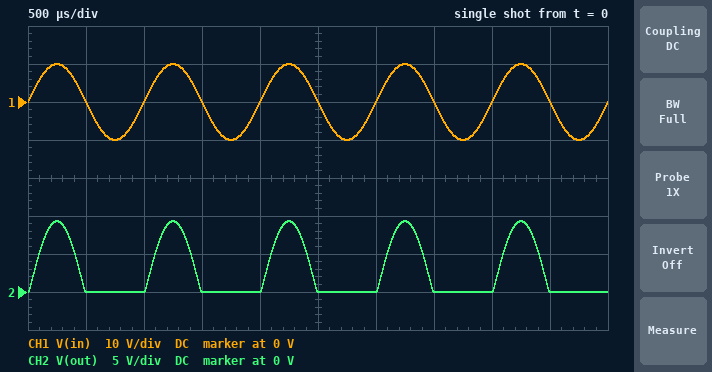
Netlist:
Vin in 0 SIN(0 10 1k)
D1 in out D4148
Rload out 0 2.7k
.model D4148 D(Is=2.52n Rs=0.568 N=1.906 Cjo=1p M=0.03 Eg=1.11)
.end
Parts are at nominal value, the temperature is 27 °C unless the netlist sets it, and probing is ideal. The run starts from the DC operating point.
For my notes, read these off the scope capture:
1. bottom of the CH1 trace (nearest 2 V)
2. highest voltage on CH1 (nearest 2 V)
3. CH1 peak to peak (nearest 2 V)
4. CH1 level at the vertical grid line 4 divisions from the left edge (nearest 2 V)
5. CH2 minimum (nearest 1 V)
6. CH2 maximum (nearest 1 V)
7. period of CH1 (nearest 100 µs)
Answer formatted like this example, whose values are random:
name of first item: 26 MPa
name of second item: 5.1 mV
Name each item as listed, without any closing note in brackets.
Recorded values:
bottom of the CH1 trace: -10 V
highest voltage on CH1: 10 V
CH1 peak to peak: 20 V
CH1 level at the vertical grid line 4 divisions from the left edge: 0 V
CH2 minimum: 0 V
CH2 maximum: 9 V
period of CH1: 1.0 ms
